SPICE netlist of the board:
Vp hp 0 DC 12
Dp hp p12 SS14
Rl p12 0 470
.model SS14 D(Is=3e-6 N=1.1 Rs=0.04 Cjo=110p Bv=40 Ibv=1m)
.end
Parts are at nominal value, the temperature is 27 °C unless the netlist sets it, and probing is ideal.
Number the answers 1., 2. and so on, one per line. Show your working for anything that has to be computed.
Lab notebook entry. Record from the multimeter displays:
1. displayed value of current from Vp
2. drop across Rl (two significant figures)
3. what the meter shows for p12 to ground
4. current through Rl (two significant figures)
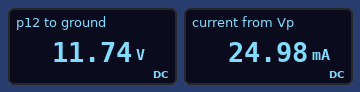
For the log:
1. 24.98 mA
2. 11.74 V = 12 V
3. 11.74 V
4. (11.74 V) / 470 Ω = 25 mA
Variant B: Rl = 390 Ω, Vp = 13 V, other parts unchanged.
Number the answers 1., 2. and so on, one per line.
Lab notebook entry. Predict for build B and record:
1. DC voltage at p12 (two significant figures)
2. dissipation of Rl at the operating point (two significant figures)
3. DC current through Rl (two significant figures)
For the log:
1. 13 V
2. 420 mW
3. 33 mA
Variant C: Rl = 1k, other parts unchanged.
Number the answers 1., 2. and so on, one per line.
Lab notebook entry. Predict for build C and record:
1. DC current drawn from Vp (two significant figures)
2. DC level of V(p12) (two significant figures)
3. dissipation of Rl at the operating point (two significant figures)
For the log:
1. 12 mA
2. 12 V
3. 140 mW
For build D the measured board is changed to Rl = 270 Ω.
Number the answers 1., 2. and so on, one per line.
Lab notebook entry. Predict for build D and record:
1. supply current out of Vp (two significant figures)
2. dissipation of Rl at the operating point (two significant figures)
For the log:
1. 43 mA
2. 510 mW
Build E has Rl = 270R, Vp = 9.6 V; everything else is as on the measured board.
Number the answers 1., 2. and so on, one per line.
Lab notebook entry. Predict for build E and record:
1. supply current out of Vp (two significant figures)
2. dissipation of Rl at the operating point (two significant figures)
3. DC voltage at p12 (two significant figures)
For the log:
1. 35 mA
2. 320 mW
3. 9.3 V
